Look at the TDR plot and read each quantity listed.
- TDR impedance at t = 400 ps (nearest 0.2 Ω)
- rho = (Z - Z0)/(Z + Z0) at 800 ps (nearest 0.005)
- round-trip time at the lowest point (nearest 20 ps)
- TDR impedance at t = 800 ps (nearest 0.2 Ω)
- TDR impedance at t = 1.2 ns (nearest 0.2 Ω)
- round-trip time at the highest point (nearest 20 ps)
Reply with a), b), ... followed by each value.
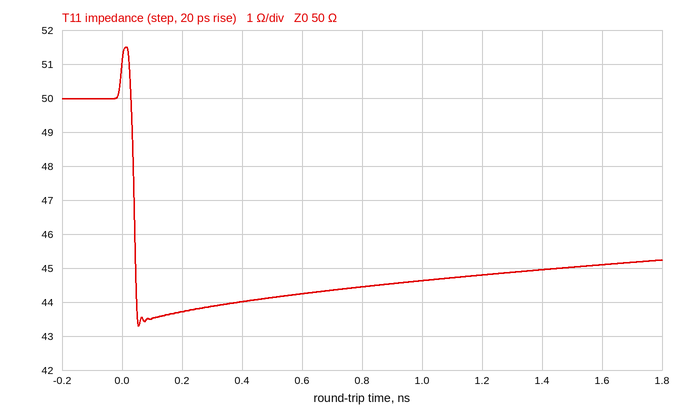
a) 44.0 Ω
b) -0.060
c) 60 ps
d) 44.4 Ω
e) 44.8 Ω
f) 20 ps
